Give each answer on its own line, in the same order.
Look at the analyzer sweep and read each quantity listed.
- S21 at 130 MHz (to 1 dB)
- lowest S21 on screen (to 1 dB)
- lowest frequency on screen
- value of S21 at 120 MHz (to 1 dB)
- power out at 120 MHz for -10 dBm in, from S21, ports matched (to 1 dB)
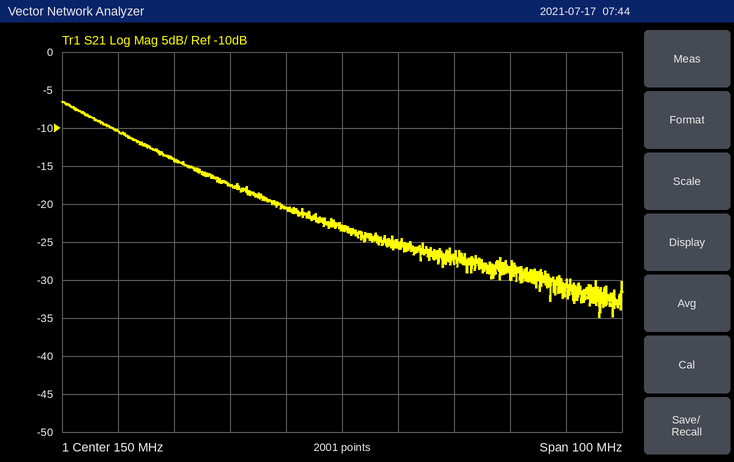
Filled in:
-18 dB
-35 dB
100 MHz
-14 dB
-24 dBm
